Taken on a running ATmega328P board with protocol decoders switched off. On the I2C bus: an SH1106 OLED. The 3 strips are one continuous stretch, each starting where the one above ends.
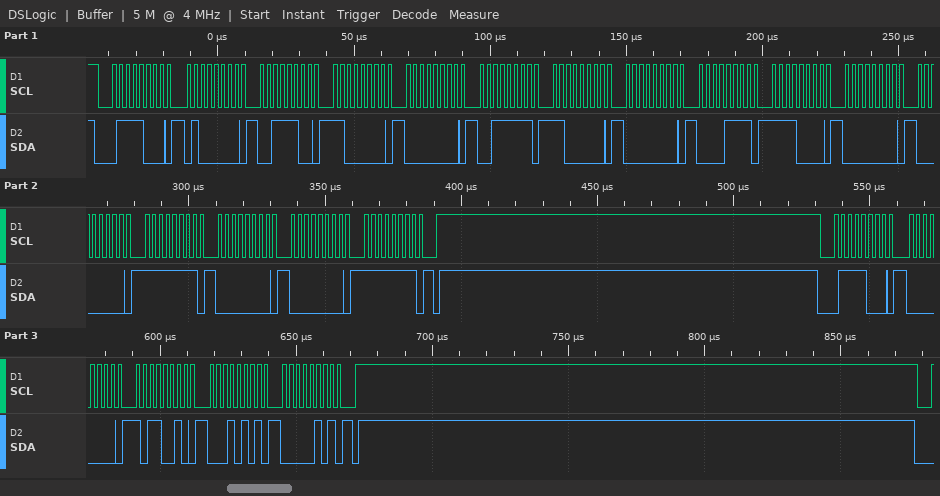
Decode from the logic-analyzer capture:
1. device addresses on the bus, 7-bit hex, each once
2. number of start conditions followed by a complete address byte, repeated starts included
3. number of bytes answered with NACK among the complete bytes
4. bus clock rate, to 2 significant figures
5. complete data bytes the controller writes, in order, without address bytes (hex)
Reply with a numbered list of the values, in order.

1. 0x3C
2. 2
3. 0
4. 400 kHz
5. 40 3C C0 00 3F C0 00 0F F0 00 00 FF 00 00 FF 00 B2 15 05
